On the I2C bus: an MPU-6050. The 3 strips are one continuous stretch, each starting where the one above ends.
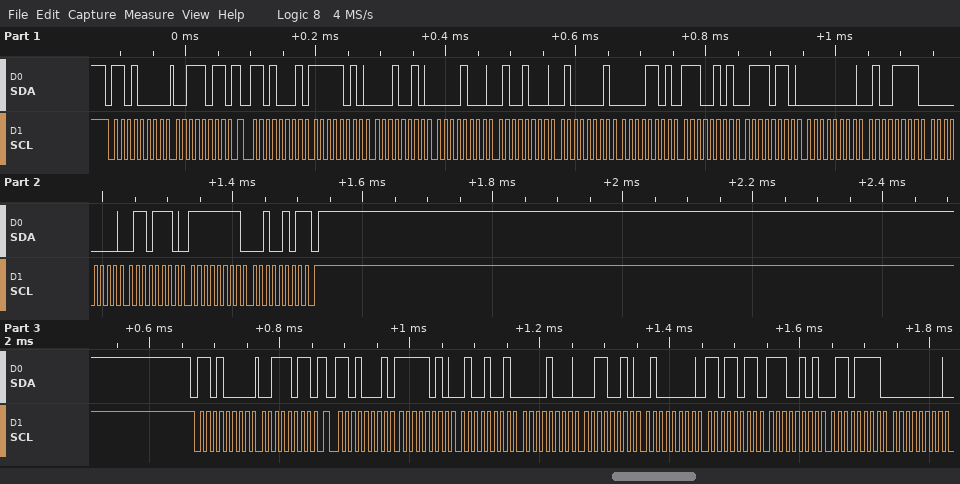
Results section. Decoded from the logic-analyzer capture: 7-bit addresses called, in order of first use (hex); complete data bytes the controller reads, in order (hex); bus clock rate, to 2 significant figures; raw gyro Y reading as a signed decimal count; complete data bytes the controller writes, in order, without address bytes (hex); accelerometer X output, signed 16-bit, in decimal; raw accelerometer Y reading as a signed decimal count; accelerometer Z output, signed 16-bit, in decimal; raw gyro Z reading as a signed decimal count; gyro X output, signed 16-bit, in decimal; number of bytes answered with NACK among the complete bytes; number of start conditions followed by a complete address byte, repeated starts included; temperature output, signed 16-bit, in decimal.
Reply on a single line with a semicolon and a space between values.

0x68; FA 12 08 48 41 0D E5 76 00 4F 00 6E FF 25 FA 49 08 32 40 DB E5 6F 00; 100 kHz; 110; 3B 3B; -1518; 2120; 16653; -219; 79; 1; 4; -6794
